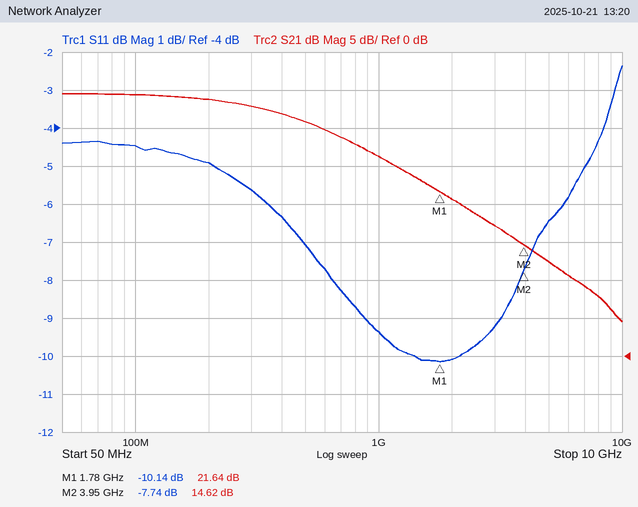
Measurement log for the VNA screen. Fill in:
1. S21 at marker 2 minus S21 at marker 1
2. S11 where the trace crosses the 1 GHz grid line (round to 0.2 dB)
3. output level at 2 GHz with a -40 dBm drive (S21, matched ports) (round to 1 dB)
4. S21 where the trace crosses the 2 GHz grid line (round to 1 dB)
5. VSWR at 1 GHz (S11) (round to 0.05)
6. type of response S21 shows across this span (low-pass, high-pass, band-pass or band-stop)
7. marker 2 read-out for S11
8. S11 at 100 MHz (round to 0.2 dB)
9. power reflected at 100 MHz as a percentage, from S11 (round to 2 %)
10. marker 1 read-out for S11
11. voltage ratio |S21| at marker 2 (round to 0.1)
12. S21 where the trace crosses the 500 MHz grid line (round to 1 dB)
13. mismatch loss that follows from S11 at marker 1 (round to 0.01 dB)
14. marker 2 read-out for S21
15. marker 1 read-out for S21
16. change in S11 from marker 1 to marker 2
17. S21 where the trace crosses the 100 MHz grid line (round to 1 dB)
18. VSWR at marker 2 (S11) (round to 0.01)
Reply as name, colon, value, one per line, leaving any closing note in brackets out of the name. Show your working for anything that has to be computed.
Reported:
S21 at marker 2 minus S21 at marker 1: 14.62 − (21.64) = -7.02 dB
S11 where the trace crosses the 1 GHz grid line: -9.4 dB
output level at 2 GHz with a -40 dBm drive (S21, matched ports): -40 dBm + (21 dB) = -19 dBm
S21 where the trace crosses the 2 GHz grid line: 21 dB
VSWR at 1 GHz (S11): |Γ| = 10^(-9.4/20) = 0.3388; VSWR = (1 + 0.3388)/(1 − 0.3388) ≈ 2.03, so 2.05 to the nearest 0.05
type of response S21 shows across this span: low-pass
marker 2 read-out for S11: -7.74 dB
S11 at 100 MHz: -4.4 dB
power reflected at 100 MHz as a percentage, from S11: 10^(-4.4/10) ≈ 36 %
marker 1 read-out for S11: -10.14 dB
voltage ratio |S21| at marker 2: 10^(14.62/20) ≈ 5.4
S21 where the trace crosses the 500 MHz grid line: 31 dB
mismatch loss that follows from S11 at marker 1: −10 log10(1 − 10^(-10.14/10)) ≈ 0.44 dB
marker 2 read-out for S21: 14.62 dB
marker 1 read-out for S21: 21.64 dB
change in S11 from marker 1 to marker 2: -7.74 − (-10.14) = 2.40 dB
S21 where the trace crosses the 100 MHz grid line: 34 dB
VSWR at marker 2 (S11): (1 + 0.4102)/(1 − 0.4102) ≈ 2.39
